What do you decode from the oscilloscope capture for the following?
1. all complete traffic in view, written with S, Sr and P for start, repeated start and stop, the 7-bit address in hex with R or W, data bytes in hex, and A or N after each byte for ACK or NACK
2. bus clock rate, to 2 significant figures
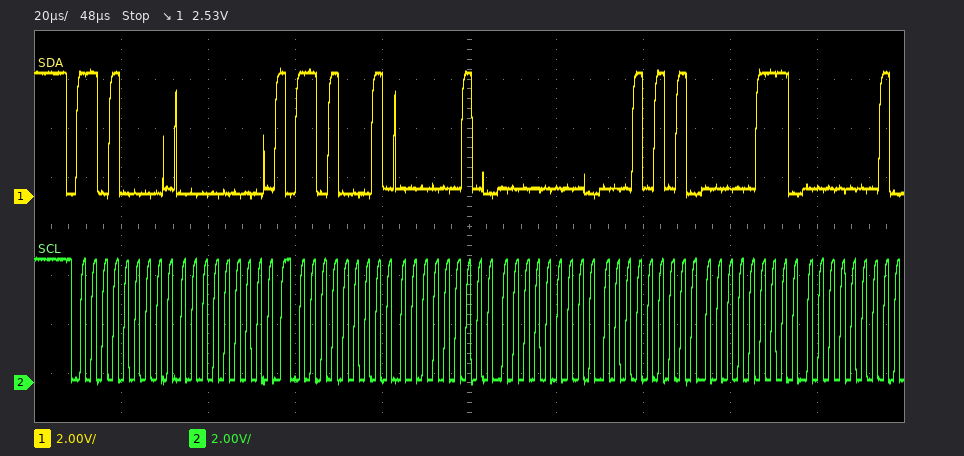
S 68W A 00 A Sr 68R A 02 A 00 A 15 A 07 A 01 A
400 kHz
